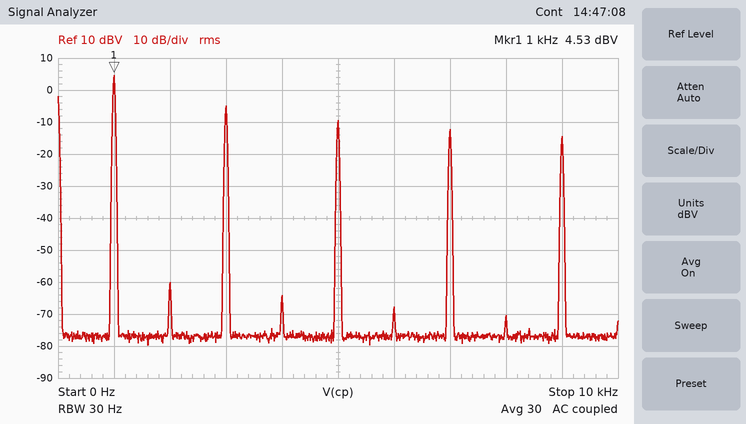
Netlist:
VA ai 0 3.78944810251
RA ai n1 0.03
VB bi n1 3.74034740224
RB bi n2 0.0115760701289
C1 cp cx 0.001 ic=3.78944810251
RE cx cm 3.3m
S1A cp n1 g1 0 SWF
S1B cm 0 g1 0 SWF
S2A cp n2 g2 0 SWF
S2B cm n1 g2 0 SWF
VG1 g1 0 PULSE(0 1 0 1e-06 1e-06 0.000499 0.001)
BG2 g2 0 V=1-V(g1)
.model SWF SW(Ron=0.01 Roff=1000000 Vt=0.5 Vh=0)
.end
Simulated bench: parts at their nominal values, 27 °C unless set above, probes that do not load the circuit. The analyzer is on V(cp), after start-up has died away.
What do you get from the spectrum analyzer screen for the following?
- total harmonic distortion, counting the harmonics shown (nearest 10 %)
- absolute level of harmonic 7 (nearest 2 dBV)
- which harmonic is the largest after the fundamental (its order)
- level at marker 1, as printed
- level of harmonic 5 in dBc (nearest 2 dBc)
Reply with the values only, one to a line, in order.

40 %
-12 dBV
3
4.53 dBV
-14 dBc
